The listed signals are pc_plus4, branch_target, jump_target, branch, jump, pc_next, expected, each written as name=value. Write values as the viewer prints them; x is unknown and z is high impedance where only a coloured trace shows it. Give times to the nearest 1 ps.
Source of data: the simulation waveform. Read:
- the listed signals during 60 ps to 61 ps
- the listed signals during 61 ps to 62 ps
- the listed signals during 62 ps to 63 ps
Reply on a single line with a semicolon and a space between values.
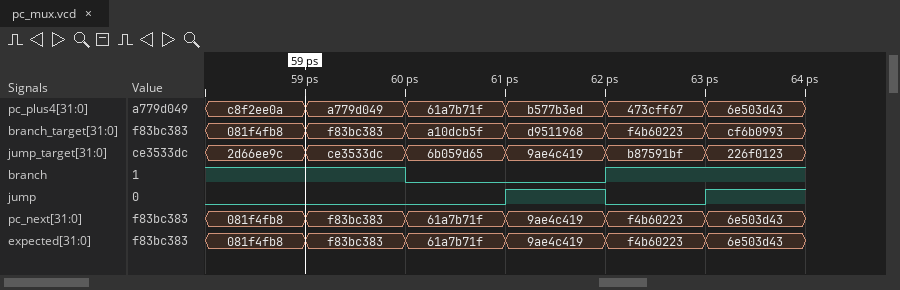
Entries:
pc_plus4=61a7b71f, branch_target=a10dcb5f, jump_target=6b059d65, branch=0, jump=0, pc_next=61a7b71f, expected=61a7b71f; pc_plus4=b577b3ed, branch_target=d9511968, jump_target=9ae4c419, branch=0, jump=1, pc_next=9ae4c419, expected=9ae4c419; pc_plus4=473cff67, branch_target=f4b60223, jump_target=b87591bf, branch=1, jump=0, pc_next=f4b60223, expected=f4b60223
